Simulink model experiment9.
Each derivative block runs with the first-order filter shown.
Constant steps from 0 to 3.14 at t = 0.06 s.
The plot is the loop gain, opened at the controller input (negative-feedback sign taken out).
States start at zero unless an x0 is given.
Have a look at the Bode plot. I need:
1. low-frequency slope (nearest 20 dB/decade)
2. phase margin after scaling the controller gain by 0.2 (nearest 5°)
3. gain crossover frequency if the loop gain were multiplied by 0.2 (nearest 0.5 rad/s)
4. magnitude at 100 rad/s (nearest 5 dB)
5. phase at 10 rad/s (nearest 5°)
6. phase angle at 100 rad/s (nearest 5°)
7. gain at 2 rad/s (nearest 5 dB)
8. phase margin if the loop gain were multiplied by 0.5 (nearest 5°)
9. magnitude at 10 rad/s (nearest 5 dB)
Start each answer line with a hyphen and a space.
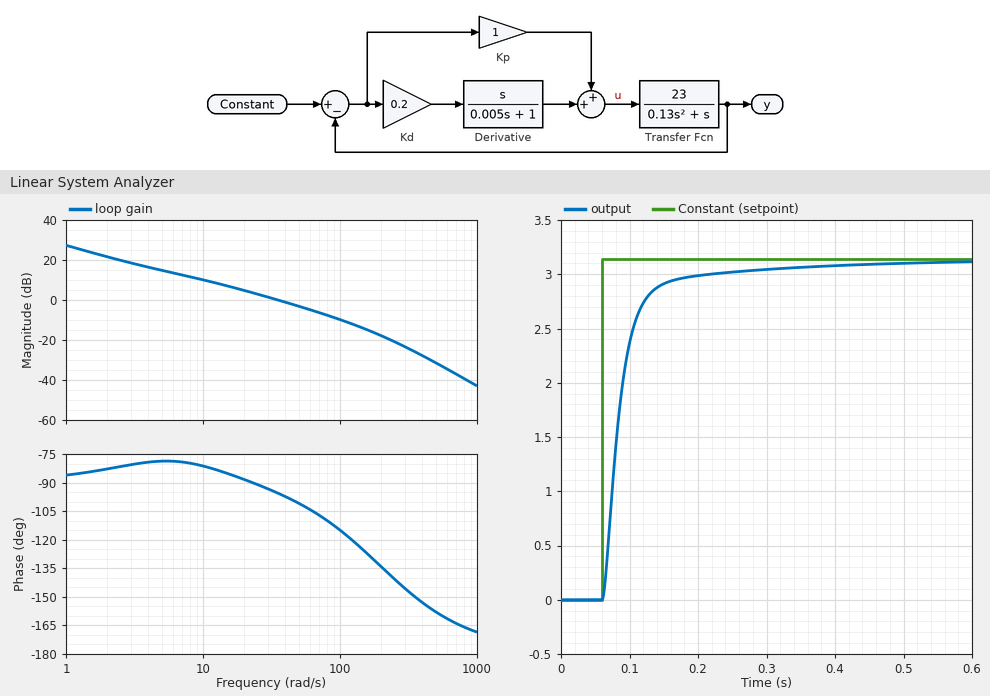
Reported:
- -20 dB/decade
- 100°
- 5.5 rad/s
- -10 dB
- -80°
- -115°
- 20 dB
- 95°
- 10 dB
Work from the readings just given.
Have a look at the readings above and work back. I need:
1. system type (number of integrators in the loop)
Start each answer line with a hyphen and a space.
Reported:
- 1
